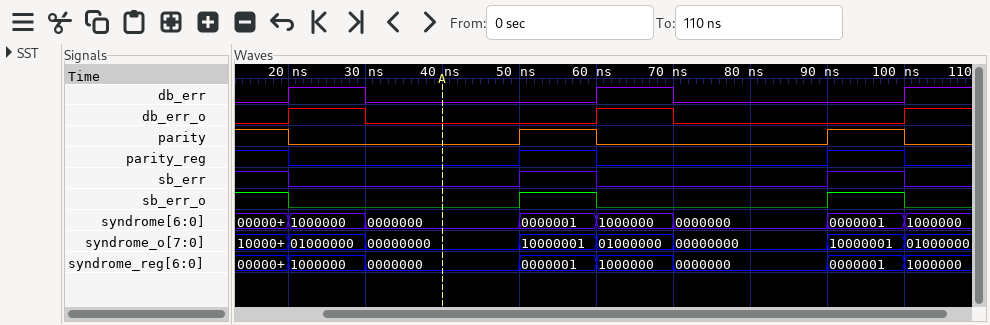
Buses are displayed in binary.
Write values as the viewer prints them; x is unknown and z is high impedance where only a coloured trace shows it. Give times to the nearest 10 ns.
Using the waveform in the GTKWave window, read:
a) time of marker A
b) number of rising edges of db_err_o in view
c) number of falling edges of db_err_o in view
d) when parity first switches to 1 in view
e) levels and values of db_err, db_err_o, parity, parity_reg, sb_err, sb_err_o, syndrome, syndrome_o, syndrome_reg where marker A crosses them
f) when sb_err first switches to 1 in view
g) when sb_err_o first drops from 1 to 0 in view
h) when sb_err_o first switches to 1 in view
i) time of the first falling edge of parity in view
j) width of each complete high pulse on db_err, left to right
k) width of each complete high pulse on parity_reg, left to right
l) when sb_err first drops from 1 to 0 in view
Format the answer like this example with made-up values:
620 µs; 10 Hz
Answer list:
40 ns; 3; 2; 50 ns; db_err=0, db_err_o=0, parity=0, parity_reg=0, sb_err=0, sb_err_o=0, syndrome=0000000, syndrome_o=00000000, syndrome_reg=0000000; 50 ns; 20 ns; 50 ns; 20 ns; 10 ns, 10 ns; 10 ns, 10 ns; 20 ns
